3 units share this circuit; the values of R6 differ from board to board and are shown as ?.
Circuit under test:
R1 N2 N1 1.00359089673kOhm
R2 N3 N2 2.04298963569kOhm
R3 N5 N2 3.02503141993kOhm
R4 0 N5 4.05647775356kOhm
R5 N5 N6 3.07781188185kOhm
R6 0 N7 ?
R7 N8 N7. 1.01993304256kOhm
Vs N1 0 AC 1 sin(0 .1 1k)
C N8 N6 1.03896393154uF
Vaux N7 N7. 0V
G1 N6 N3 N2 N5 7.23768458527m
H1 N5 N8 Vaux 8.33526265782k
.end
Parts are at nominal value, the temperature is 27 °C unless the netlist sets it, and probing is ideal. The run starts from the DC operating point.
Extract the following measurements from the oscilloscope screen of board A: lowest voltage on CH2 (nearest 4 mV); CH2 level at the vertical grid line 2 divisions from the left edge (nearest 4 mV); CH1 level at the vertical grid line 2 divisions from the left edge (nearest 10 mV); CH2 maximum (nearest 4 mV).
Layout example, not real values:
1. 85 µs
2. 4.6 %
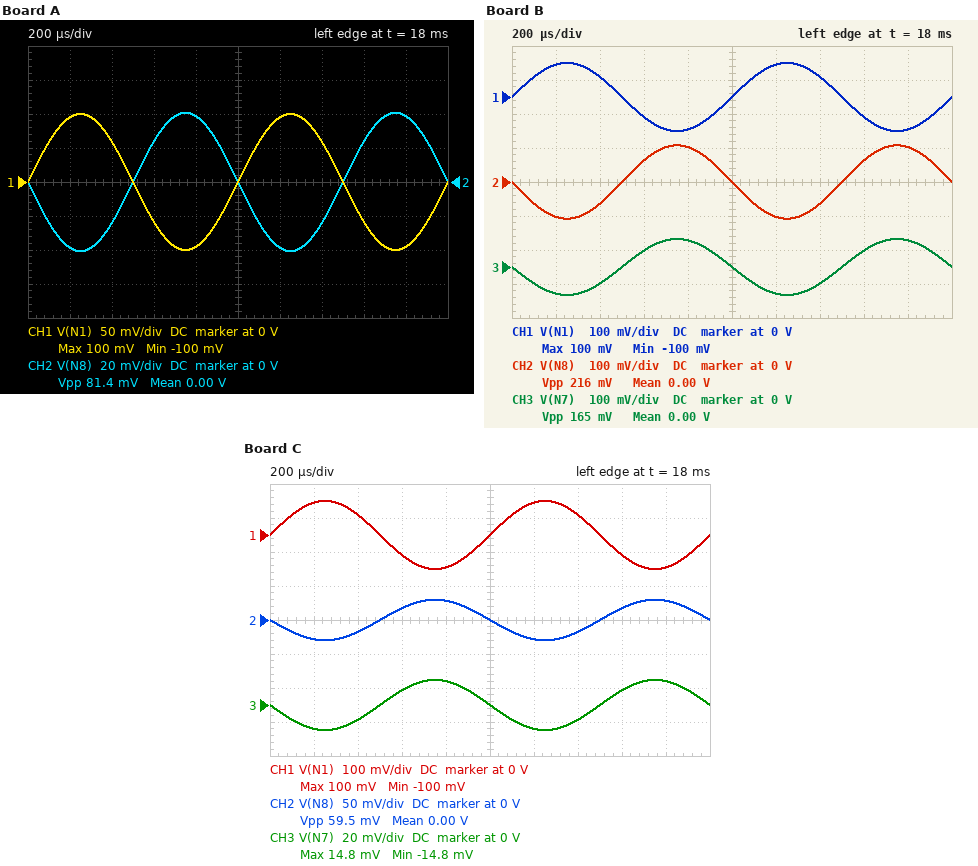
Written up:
1. -40 mV
2. -24 mV
3. 60 mV
4. 40 mV
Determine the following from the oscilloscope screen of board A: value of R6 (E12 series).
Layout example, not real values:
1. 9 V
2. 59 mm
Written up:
1. 1.5 kΩ
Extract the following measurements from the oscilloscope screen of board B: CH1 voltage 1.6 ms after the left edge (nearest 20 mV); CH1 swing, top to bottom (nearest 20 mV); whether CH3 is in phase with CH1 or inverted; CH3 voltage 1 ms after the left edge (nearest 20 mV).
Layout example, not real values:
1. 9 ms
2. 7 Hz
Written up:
1. -60 mV
2. 200 mV
3. inverted
4. 0 V
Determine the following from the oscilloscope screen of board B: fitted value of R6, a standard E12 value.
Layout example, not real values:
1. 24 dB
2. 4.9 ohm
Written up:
1. 3.3 kΩ
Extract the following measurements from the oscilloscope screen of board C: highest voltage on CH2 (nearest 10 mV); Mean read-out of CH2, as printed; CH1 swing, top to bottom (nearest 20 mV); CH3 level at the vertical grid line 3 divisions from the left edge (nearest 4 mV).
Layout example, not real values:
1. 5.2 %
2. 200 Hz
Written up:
1. 30 mV
2. 0.00 V
3. 200 mV
4. 8 mV
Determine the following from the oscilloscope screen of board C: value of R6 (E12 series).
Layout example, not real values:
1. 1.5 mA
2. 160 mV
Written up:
1. 1 kΩ
